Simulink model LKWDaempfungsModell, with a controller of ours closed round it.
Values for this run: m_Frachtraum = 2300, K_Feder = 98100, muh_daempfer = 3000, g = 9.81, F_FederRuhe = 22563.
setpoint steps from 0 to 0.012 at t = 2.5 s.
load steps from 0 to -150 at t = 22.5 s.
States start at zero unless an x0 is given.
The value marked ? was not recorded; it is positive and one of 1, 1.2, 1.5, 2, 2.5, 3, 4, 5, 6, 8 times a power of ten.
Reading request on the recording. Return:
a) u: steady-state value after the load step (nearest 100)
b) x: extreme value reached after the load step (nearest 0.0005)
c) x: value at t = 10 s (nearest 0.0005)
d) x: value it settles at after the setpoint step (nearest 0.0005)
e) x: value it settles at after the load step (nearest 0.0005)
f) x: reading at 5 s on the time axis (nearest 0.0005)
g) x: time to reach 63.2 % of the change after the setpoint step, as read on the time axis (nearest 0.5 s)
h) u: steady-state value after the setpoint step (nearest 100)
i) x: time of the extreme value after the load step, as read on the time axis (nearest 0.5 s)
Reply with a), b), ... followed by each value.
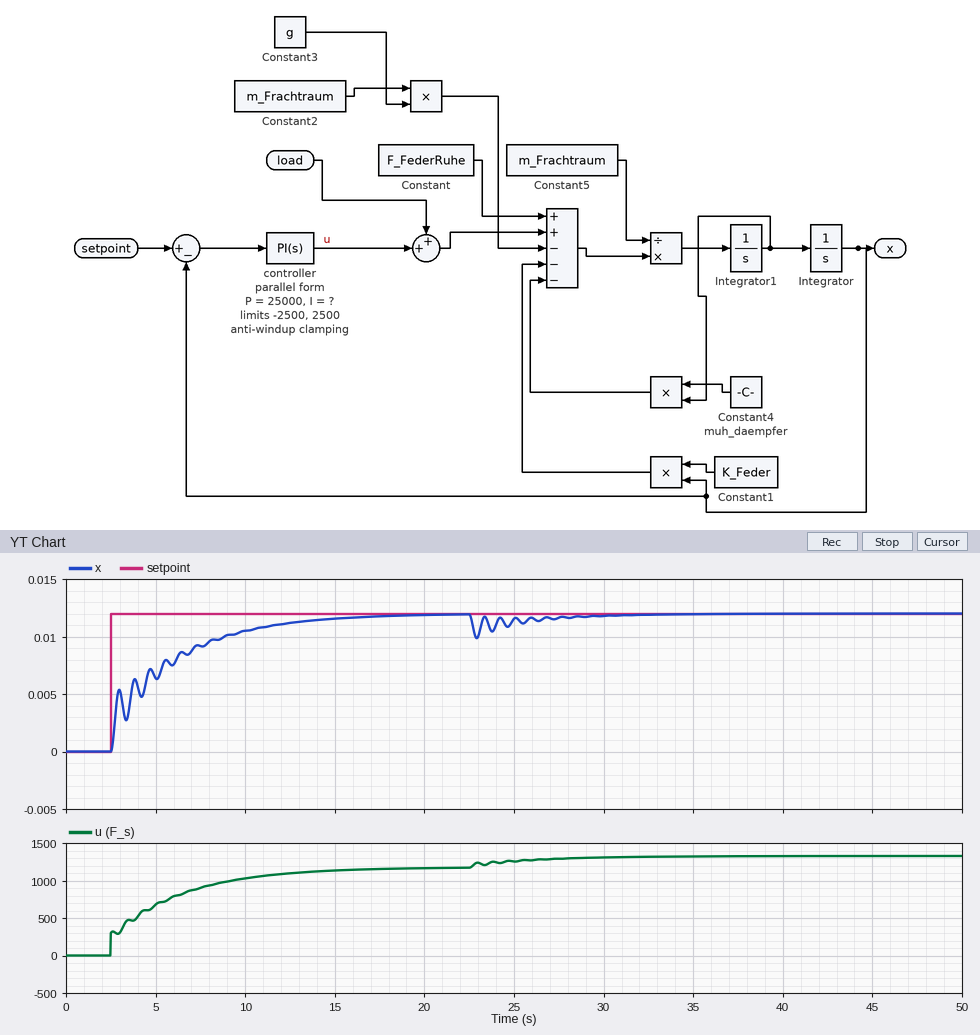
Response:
a) 1300
b) 0.0100
c) 0.0105
d) 0.0120
e) 0.0120
f) 0.0065
g) 5.5 s
h) 1200
i) 23.0 s
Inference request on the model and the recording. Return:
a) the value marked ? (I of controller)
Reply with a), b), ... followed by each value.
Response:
a) 30000
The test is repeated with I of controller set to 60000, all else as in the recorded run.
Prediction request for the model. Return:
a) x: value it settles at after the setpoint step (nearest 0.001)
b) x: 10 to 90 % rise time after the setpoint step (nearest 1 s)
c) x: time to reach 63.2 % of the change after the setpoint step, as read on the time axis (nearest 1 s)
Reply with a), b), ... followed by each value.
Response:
a) 0.012
b) 4 s
c) 4 s
